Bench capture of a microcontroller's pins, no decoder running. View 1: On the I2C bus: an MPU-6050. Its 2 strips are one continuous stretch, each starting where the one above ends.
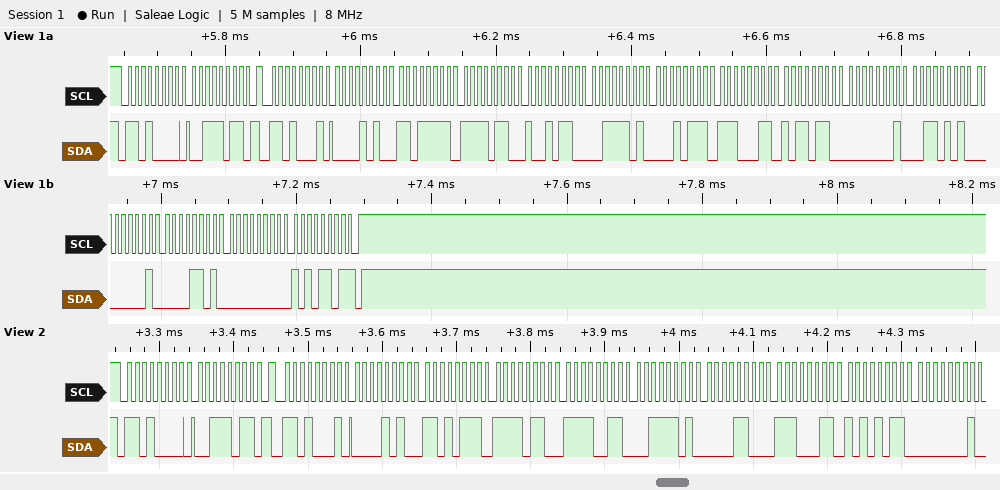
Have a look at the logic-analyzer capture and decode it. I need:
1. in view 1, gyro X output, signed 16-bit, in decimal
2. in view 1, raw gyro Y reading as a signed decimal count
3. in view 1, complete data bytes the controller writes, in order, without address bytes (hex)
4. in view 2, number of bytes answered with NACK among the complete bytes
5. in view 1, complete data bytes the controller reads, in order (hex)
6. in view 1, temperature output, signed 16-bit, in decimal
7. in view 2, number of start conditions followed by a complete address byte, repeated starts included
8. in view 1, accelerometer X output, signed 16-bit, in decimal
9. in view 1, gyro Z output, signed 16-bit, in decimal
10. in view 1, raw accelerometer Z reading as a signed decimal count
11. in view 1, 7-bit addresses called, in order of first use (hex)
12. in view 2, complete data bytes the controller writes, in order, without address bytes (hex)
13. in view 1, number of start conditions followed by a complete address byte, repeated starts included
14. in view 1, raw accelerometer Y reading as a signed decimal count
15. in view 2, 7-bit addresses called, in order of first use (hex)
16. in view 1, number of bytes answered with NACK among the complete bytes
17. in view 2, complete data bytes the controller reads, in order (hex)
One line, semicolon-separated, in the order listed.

309; 269; 3B; 0; 0A DF F6 96 3D 17 E3 B6 01 35 01 0D 00 AD; -7242; 2; 2783; 173; 15639; 0x68; 3B; 2; -2410; 0x68; 1; 0A D7 F6 F3 3D 0C E3 AB 01
